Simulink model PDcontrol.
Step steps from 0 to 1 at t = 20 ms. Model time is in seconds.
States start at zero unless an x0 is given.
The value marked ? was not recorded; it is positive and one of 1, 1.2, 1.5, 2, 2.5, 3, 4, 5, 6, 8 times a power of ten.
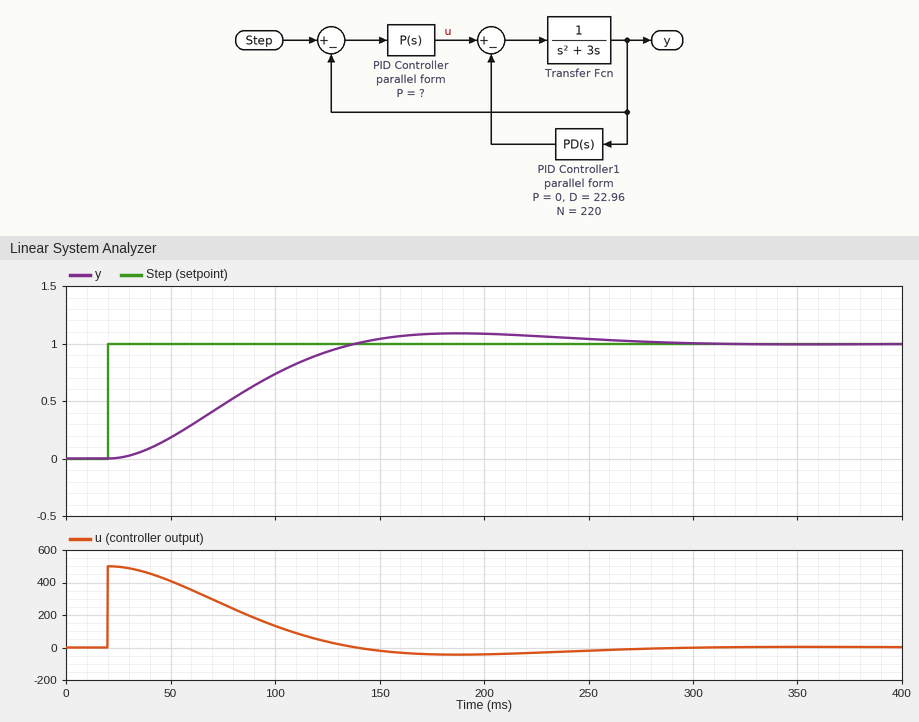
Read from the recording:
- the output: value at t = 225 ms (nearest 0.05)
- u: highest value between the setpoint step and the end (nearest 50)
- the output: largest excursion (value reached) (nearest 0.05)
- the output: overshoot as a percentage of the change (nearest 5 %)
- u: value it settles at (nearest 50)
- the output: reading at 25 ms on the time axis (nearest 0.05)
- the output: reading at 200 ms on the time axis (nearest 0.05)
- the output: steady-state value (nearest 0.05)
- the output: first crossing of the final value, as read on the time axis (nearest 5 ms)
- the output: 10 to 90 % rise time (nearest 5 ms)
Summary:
1.05
500
1.10
10 %
0
0.00
1.10
1.00
140 ms
80 ms
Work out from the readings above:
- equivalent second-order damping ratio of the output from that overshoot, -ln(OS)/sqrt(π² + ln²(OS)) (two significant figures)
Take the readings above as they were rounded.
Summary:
0.59
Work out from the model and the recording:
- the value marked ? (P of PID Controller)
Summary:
500
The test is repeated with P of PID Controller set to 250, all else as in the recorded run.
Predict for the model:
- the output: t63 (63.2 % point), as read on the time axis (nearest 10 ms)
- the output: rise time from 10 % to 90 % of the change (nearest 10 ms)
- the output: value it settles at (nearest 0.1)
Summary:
140 ms
160 ms
1.0
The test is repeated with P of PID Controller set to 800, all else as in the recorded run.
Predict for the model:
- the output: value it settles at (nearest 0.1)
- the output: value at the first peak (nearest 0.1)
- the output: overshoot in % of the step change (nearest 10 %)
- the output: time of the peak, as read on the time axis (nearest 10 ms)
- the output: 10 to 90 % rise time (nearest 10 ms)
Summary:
1.0
1.2
20 %
140 ms
50 ms
